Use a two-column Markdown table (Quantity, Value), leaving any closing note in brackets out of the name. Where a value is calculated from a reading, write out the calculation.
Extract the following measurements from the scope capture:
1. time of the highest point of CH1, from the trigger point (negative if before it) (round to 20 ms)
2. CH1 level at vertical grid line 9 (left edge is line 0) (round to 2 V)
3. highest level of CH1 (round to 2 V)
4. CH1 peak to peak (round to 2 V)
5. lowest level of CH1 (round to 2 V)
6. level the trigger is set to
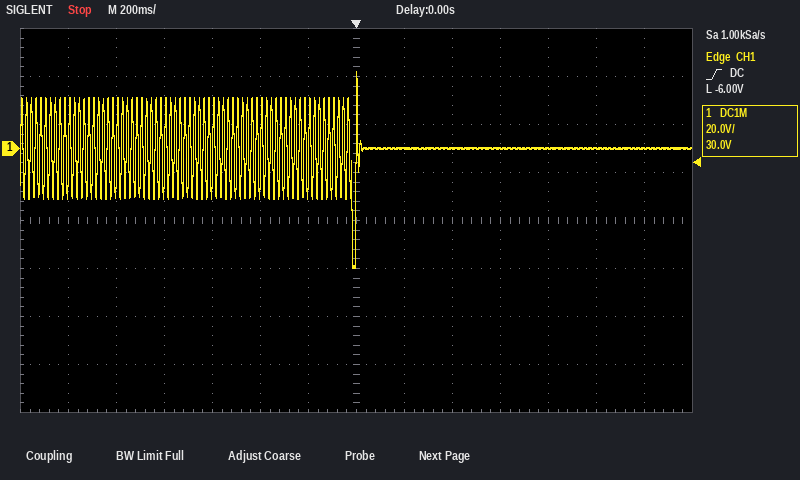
| Quantity | Value |
|---|---|
| time of the highest point of CH1, from the trigger point (negative if before it) | 0 ms |
| CH1 level at vertical grid line 9 (left edge is line 0) | 0 V |
| highest level of CH1 | 32 V |
| CH1 peak to peak | 32 V − (-50 V) = 82 V |
| lowest level of CH1 | -50 V |
| level the trigger is set to | -6.00 V |
